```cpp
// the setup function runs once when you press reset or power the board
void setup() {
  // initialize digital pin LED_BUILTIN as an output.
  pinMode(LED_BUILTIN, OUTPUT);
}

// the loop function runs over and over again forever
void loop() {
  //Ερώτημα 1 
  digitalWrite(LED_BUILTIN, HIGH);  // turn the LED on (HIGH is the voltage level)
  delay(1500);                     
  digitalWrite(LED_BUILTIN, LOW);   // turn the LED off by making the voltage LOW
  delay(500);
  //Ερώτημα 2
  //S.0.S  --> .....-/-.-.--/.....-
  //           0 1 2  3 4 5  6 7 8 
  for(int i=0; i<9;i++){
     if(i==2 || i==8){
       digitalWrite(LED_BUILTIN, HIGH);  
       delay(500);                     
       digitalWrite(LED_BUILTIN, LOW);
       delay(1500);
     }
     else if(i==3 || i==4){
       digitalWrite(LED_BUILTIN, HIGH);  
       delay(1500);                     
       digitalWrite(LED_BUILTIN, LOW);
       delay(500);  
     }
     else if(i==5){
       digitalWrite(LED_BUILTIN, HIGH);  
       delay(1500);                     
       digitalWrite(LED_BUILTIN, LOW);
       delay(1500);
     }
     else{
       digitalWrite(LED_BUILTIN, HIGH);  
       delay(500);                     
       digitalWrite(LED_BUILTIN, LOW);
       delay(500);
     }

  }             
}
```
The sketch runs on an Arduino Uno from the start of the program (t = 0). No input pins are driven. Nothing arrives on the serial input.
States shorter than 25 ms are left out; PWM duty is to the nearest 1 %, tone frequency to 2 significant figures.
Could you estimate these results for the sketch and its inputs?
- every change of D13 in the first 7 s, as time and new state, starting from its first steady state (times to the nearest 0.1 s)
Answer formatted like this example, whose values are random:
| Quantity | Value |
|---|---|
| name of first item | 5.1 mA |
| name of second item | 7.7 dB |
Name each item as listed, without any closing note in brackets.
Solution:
| Quantity | Value |
|---|---|
| every change of D13 in the first 7 s, as time and new state, starting from its first steady state | 0 s high; 1.5 s low; 2 s high; 2.5 s low; 3 s high; 3.5 s low; 4 s high; 4.5 s low; 6 s high |
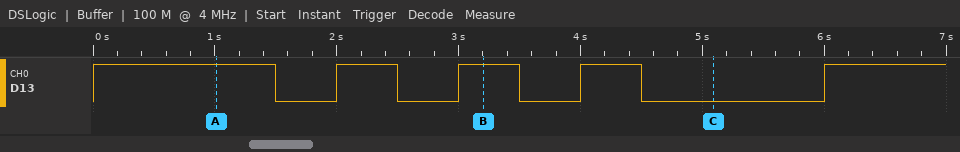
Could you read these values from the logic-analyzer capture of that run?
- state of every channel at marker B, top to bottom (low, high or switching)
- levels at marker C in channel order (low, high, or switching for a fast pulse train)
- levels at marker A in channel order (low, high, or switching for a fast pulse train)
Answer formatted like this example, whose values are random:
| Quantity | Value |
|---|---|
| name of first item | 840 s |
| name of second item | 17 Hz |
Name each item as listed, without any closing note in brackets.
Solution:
| Quantity | Value |
|---|---|
| state of every channel at marker B, top to bottom | D13 high |
| levels at marker C in channel order | D13 low |
| levels at marker A in channel order | D13 high |
